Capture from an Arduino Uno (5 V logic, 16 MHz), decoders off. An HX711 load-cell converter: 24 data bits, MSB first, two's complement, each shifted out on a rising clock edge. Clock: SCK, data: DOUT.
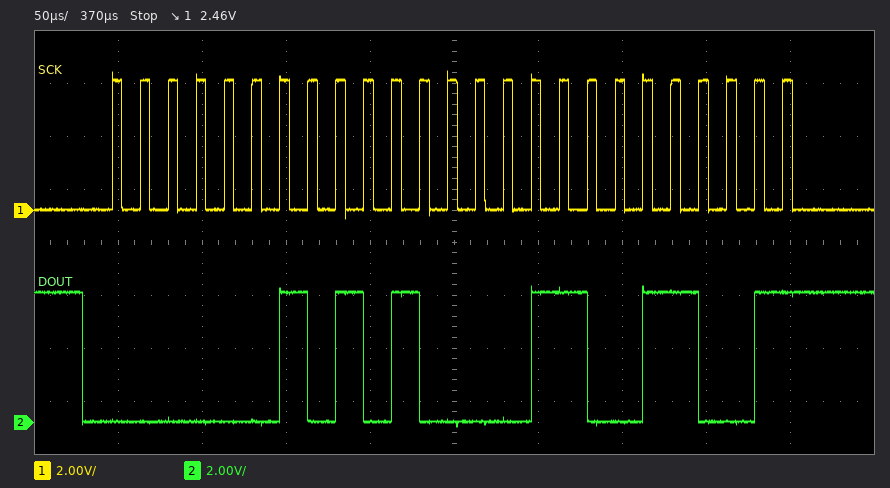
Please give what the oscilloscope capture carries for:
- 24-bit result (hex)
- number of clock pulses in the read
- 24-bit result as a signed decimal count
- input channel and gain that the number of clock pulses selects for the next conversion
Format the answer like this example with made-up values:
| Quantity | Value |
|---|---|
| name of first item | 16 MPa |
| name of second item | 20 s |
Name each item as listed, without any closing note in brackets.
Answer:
| Quantity | Value |
|---|---|
| 24-bit result | 0x02A199 |
| number of clock pulses in the read | 25 |
| 24-bit result as a signed decimal count | 172441 |
| input channel and gain that the number of clock pulses selects for the next conversion | channel A, gain 128 |
